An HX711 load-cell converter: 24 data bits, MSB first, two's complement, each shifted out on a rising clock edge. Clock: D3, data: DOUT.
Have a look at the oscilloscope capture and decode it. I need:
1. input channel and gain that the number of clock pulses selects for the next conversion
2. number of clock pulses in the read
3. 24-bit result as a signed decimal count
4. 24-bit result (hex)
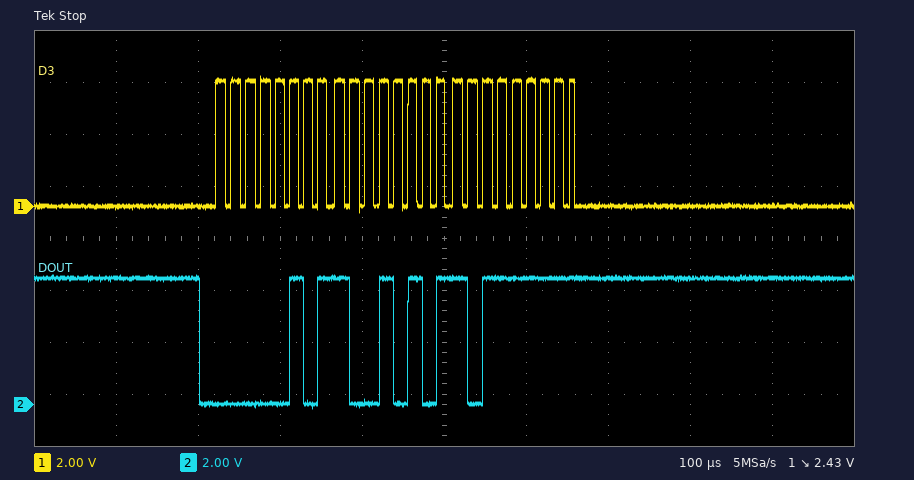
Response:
channel A, gain 128
25
366015
0x0595BF
